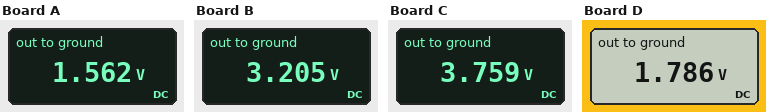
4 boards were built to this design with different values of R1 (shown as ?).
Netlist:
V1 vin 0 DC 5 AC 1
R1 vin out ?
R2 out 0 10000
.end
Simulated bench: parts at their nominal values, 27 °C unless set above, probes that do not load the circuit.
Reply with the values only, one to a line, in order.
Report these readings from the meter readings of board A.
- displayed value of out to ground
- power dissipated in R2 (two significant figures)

1.562 V
240 µW
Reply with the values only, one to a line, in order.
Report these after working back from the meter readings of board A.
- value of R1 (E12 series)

22 kΩ
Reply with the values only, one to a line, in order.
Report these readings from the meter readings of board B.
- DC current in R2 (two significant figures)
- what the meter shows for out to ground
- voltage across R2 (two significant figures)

320 µA
3.205 V
3.2 V
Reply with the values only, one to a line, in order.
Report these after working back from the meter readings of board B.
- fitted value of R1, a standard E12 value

5.6 kΩ
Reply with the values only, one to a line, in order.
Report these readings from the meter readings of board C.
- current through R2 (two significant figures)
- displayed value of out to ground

380 µA
3.759 V
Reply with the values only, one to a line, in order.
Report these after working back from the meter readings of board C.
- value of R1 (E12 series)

3.3 kΩ
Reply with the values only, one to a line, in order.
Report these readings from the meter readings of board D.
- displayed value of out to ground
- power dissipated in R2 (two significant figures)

1.786 V
320 µW
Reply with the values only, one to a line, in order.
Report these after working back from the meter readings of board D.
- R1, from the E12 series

18 kΩ
